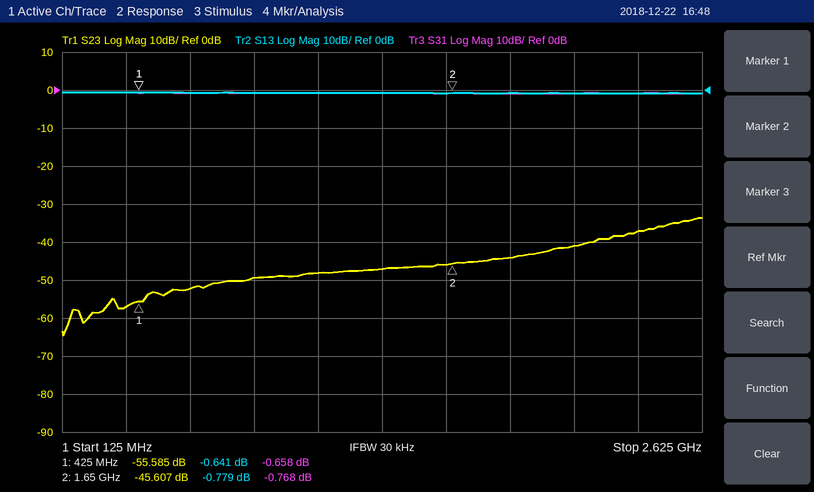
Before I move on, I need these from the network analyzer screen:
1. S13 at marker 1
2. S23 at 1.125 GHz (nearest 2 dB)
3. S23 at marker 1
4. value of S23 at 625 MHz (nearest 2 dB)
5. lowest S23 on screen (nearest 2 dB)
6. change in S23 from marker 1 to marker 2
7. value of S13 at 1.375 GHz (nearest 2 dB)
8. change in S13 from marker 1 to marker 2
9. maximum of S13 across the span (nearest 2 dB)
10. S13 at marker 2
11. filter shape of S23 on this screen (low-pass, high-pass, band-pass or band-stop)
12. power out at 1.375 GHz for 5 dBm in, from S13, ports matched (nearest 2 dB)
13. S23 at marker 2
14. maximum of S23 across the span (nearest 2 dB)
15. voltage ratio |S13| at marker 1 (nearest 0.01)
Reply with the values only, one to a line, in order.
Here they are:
-0.641 dB
-48 dB
-55.585 dB
-52 dB
-64 dB
9.978 dB
0 dB
-0.138 dB
0 dB
-0.779 dB
high-pass
4 dBm
-45.607 dB
-34 dB
0.93
